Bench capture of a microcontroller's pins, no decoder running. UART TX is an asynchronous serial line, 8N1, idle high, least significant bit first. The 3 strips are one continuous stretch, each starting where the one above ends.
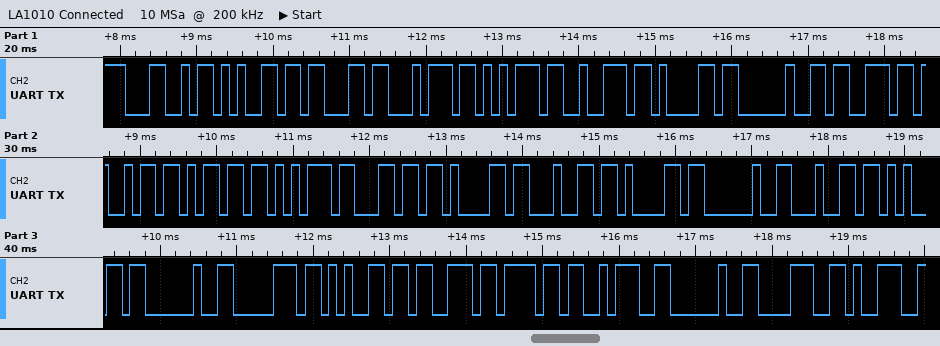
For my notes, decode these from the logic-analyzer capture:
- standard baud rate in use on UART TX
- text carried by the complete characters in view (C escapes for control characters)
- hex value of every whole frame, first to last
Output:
9600 baud
"Lectura simulada de peso: 89"
4C 65 63 74 75 72 61 20 73 69 6D 75 6C 61 64 61 20 64 65 20 70 65 73 6F 3A 20 38 39
